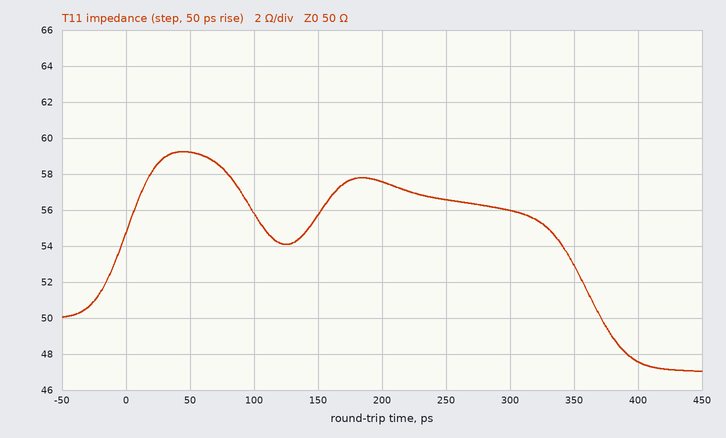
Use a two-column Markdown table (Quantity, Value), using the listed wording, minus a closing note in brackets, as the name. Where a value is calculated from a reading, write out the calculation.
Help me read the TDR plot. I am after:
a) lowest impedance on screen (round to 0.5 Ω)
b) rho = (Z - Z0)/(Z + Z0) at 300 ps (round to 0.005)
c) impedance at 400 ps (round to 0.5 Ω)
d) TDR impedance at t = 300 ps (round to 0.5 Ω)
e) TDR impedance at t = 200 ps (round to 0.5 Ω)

| Quantity | Value |
|---|---|
| lowest impedance on screen | 47.0 Ω |
| rho = (Z - Z0)/(Z + Z0) at 300 ps | (56 − 50)/(56 + 50) ≈ +0.0566, so +0.055 to the nearest 0.005 |
| impedance at 400 ps | 47.5 Ω |
| TDR impedance at t = 300 ps | 56.0 Ω |
| TDR impedance at t = 200 ps | 57.5 Ω |
